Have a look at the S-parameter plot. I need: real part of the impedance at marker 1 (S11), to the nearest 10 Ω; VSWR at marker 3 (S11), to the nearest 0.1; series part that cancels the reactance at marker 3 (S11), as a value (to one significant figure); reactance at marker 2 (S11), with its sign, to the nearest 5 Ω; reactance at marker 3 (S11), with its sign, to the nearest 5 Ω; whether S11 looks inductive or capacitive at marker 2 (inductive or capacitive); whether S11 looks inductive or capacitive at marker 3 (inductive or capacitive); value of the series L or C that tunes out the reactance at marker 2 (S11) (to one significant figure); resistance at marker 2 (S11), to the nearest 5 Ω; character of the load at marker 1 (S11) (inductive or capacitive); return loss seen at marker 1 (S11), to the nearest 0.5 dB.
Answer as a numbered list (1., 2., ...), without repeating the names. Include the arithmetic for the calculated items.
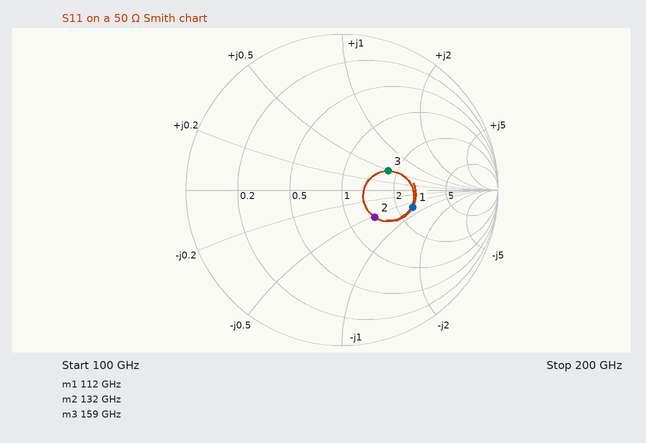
1. 130 Ω
2. 1.9
3. C = 1/(2π × 159 GHz × 25 Ω) ≈ 40 fF
4. -25 Ω
5. +25 Ω
6. capacitive
7. inductive
8. L = 25 Ω/(2π × 132 GHz) ≈ 30 pH
9. 70 Ω
10. capacitive
11. 6.5 dB
